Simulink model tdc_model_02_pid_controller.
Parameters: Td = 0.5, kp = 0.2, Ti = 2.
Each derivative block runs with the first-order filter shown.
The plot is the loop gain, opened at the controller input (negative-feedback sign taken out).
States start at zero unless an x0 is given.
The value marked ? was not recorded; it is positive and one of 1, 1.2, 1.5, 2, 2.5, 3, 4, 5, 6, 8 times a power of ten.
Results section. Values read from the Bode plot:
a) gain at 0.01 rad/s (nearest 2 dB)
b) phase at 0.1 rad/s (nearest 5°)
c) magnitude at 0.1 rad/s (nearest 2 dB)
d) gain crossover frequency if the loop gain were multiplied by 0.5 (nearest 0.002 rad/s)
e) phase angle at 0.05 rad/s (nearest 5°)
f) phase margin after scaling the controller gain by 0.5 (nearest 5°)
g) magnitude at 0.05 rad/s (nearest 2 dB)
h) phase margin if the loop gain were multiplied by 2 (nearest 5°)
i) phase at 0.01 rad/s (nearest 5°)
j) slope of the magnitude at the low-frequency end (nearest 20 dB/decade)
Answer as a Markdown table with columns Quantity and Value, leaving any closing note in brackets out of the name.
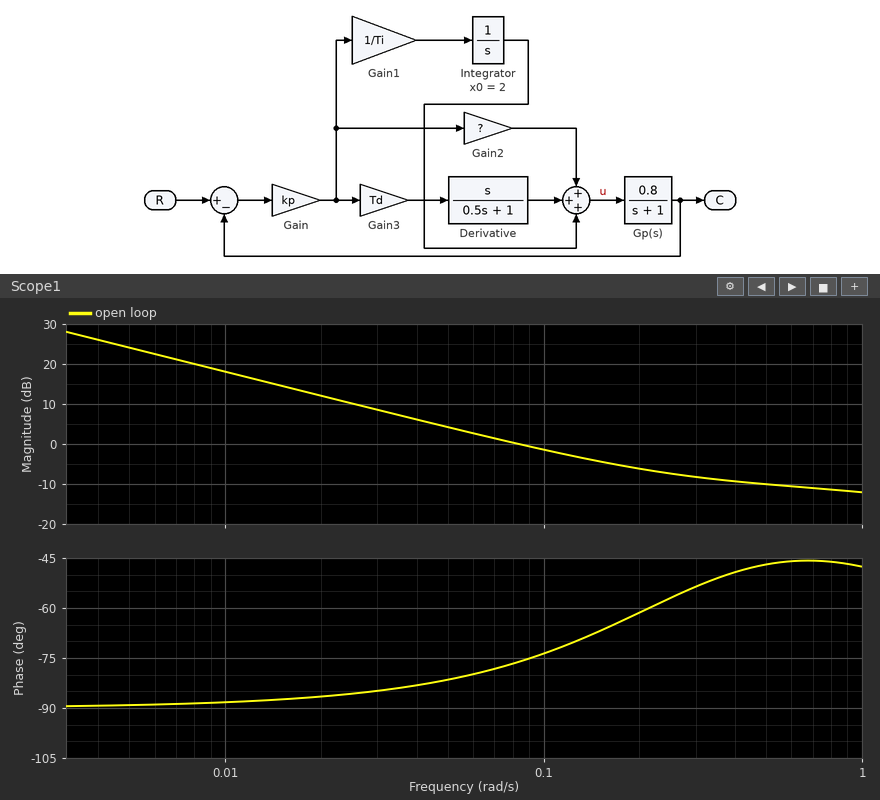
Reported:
| Quantity | Value |
|---|---|
| gain at 0.01 rad/s | 18 dB |
| phase at 0.1 rad/s | -75° |
| magnitude at 0.1 rad/s | -2 dB |
| gain crossover frequency if the loop gain were multiplied by 0.5 | 0.040 rad/s |
| phase angle at 0.05 rad/s | -80° |
| phase margin after scaling the controller gain by 0.5 | 95° |
| magnitude at 0.05 rad/s | 4 dB |
| phase margin if the loop gain were multiplied by 2 | 120° |
| phase at 0.01 rad/s | -90° |
| slope of the magnitude at the low-frequency end | -20 dB/decade |
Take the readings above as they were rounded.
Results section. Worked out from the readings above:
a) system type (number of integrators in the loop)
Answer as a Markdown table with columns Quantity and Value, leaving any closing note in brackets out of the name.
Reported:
| Quantity | Value |
|---|---|
| system type | 1 |
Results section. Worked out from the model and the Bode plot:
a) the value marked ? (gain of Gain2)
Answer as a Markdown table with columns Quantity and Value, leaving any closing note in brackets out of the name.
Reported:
| Quantity | Value |
|---|---|
| the value marked ? | 2 |
